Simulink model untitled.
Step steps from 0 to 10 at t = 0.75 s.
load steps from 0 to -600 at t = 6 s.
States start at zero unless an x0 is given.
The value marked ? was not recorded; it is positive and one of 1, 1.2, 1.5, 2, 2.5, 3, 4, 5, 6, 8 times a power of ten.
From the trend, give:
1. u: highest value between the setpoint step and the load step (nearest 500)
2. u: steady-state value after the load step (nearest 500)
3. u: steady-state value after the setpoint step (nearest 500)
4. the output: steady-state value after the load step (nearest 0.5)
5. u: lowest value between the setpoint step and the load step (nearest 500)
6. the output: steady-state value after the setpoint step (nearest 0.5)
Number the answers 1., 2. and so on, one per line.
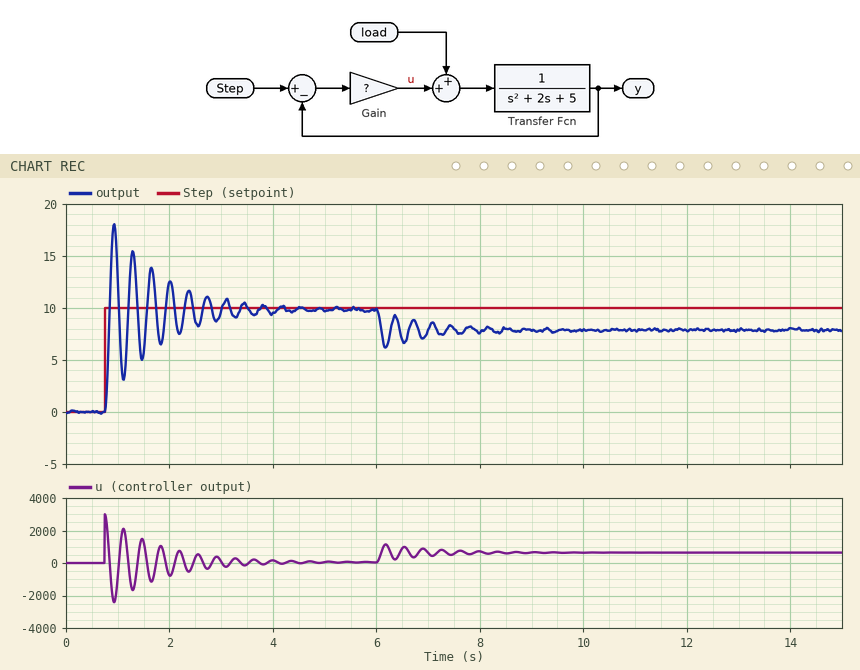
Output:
1. 3000
2. 500
3. 0
4. 8.0
5. -2500
6. 10.0
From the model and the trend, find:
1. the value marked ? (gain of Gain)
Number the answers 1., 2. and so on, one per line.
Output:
1. 300
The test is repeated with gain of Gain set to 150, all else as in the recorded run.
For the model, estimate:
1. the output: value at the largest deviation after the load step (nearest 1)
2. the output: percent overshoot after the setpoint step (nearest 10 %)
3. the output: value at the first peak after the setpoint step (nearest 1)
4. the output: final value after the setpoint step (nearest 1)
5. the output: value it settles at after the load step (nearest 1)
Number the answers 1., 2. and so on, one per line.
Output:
1. 3
2. 80 %
3. 17
4. 10
5. 6
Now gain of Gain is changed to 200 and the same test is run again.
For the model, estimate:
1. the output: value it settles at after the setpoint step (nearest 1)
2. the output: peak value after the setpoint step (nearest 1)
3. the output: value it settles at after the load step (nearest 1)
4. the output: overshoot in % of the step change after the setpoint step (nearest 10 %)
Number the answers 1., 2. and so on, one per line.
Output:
1. 10
2. 18
3. 7
4. 80 %
